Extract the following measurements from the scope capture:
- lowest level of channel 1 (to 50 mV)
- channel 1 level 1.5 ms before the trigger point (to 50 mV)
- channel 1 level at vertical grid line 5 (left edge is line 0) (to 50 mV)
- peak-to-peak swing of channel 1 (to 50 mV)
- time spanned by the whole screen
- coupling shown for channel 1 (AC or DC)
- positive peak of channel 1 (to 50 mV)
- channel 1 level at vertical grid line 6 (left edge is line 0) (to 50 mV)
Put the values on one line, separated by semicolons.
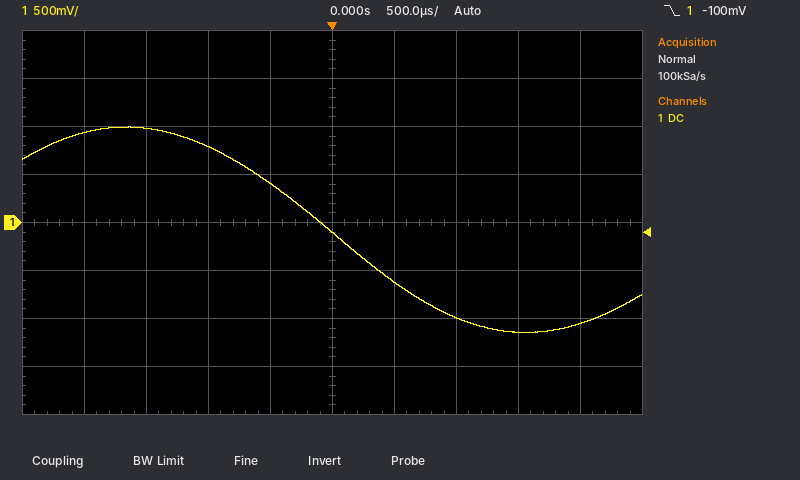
-1.15 V; 1.00 V; -100 mV; 2.15 V; 5 ms; DC; 1.00 V; -600 mV
